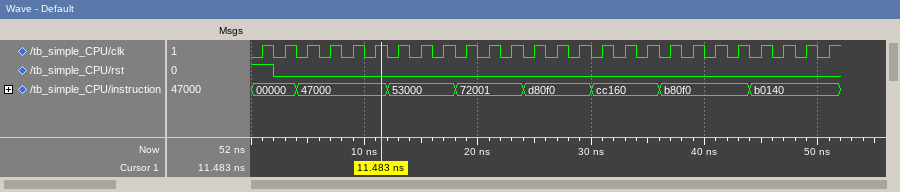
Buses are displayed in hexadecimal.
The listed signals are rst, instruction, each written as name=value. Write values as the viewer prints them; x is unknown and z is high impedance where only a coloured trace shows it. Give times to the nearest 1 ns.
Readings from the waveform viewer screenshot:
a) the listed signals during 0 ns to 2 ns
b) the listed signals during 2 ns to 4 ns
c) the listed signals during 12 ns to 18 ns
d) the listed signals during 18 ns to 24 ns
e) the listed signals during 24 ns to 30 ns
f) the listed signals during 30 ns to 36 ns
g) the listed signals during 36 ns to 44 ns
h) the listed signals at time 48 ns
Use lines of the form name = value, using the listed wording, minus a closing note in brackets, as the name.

the listed signals during 0 ns to 2 ns = rst=1, instruction=00000
the listed signals during 2 ns to 4 ns = rst=0, instruction=00000
the listed signals during 12 ns to 18 ns = rst=0, instruction=53000
the listed signals during 18 ns to 24 ns = rst=0, instruction=72001
the listed signals during 24 ns to 30 ns = rst=0, instruction=d80f0
the listed signals during 30 ns to 36 ns = rst=0, instruction=cc160
the listed signals during 36 ns to 44 ns = rst=0, instruction=b80f0
the listed signals at time 48 ns = rst=0, instruction=b0140
